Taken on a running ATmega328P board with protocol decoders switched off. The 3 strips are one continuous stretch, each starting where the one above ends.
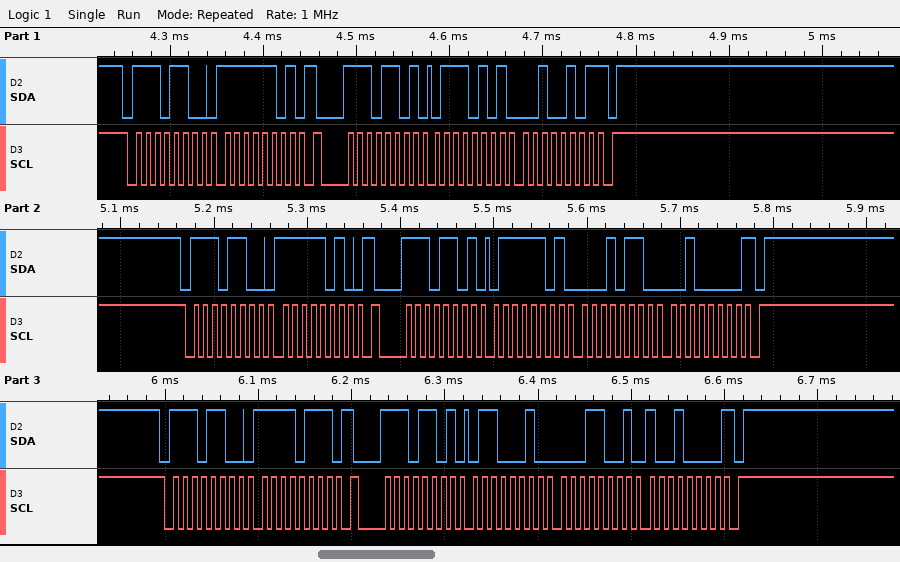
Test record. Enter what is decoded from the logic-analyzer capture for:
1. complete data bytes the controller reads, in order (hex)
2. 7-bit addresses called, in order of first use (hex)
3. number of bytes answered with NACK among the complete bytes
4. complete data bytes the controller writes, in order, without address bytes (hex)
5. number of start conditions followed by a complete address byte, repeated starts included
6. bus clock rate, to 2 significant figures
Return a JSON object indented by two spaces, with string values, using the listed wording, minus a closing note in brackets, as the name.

{
  "complete data bytes the controller reads, in order": "75 25 7D 16 20 62 19 90",
  "7-bit addresses called, in order of first use": "0x76",
  "number of bytes answered with NACK among the complete bytes": "3",
  "complete data bytes the controller writes, in order, without address bytes": "FD FA F7",
  "number of start conditions followed by a complete address byte, repeated starts included": "6",
  "bus clock rate, to 2 significant figures": "100 kHz"
}
